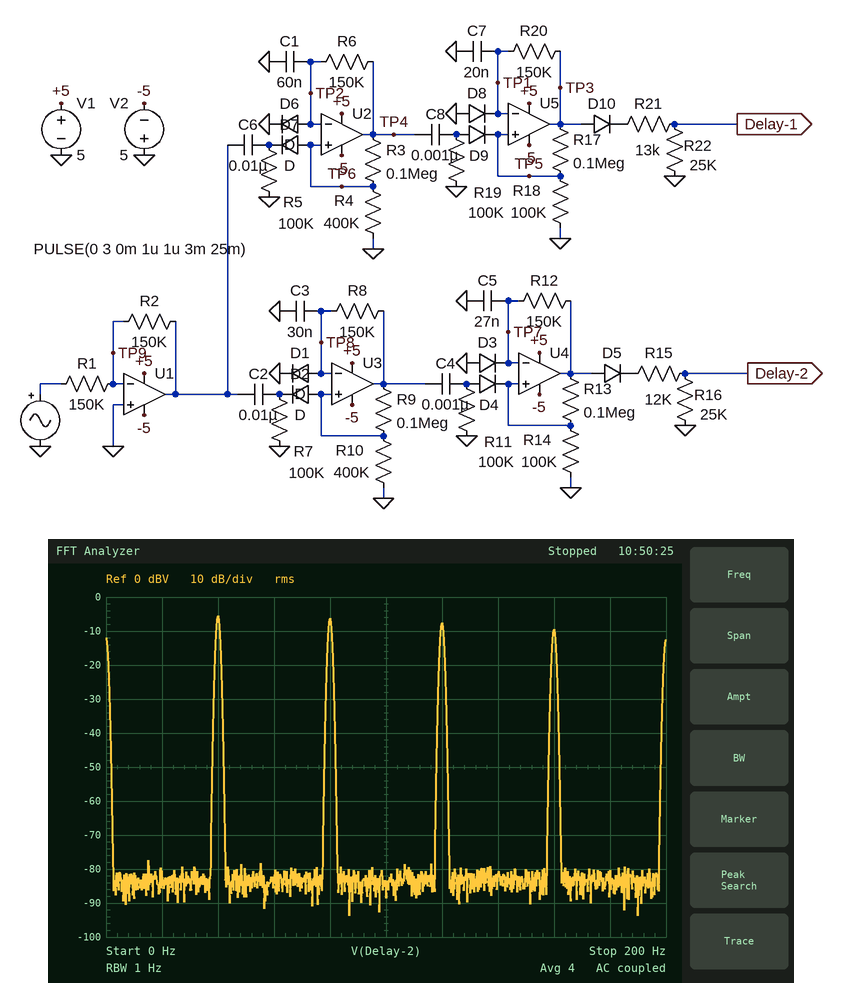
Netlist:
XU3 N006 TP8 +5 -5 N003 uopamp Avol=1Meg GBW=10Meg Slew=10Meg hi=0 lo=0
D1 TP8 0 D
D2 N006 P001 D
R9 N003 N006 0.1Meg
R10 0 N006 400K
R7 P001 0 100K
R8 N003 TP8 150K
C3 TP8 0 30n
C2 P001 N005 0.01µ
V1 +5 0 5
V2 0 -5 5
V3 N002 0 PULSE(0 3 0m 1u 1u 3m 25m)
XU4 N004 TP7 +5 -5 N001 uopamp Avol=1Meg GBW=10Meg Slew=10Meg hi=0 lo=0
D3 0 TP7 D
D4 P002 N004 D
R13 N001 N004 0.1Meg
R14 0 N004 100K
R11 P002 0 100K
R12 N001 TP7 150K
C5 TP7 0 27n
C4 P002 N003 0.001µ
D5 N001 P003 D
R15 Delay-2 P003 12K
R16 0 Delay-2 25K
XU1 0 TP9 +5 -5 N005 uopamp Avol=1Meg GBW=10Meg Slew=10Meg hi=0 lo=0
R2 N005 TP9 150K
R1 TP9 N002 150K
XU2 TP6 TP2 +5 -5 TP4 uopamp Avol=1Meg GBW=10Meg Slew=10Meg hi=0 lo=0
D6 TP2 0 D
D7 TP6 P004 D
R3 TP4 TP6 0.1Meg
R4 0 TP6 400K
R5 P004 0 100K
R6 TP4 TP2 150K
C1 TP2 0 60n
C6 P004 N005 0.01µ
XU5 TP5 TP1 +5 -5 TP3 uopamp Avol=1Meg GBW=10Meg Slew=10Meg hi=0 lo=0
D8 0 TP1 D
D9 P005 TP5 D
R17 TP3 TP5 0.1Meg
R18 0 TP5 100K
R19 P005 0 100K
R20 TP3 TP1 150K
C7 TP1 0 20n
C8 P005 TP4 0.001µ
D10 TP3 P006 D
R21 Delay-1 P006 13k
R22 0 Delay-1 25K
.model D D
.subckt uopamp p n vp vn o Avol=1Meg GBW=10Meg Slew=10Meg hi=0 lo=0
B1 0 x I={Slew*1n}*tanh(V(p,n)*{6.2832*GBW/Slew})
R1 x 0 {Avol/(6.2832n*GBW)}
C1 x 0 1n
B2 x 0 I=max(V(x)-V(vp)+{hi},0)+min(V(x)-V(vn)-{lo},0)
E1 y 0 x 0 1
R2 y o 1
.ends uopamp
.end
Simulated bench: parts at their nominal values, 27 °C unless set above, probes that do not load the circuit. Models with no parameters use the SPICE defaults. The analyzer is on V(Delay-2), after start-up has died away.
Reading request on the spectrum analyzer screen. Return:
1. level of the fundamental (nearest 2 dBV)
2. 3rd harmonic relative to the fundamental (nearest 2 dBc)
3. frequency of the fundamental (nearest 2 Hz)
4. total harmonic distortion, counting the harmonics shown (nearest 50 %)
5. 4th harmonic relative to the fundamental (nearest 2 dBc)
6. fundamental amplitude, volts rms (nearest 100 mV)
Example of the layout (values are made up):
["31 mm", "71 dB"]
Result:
["-6 dBV", "-2 dBc", "40 Hz", "150 %", "-4 dBc", "500 mV"]
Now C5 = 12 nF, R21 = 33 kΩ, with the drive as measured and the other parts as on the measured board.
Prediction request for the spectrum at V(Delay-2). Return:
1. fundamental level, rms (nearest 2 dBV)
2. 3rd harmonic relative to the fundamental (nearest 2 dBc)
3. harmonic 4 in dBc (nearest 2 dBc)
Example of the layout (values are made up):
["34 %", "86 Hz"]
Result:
["-12 dBV", "0 dBc", "0 dBc"]
